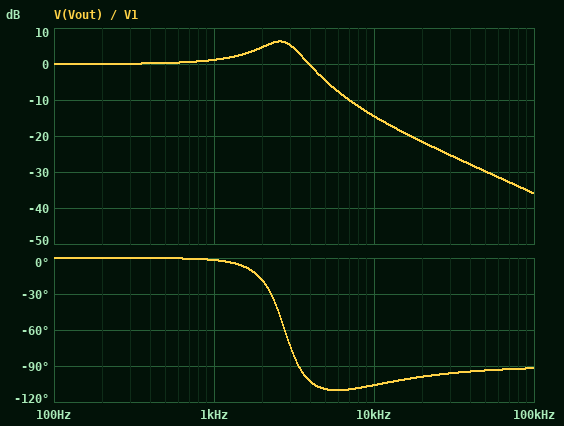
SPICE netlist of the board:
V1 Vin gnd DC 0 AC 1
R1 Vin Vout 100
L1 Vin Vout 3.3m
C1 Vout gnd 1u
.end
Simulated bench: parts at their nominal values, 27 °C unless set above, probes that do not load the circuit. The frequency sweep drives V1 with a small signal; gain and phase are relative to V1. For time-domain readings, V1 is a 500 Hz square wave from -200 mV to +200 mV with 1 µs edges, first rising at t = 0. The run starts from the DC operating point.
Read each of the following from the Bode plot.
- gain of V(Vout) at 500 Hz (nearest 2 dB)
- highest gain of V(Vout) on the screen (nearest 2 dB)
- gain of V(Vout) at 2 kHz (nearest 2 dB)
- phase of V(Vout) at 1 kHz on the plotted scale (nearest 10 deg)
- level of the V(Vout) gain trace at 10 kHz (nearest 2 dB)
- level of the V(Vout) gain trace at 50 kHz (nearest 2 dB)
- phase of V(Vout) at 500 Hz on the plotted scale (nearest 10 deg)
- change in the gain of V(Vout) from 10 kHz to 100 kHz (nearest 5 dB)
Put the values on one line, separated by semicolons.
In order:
0 dB; 6 dB; 4 dB; 0 deg; -14 dB; -30 dB; 0 deg; -20 dB
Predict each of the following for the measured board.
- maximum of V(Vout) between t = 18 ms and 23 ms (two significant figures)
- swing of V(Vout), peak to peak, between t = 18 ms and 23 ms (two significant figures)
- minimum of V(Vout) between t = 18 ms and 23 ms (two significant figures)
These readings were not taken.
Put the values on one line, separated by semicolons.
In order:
390 mV; 770 mV; -390 mV
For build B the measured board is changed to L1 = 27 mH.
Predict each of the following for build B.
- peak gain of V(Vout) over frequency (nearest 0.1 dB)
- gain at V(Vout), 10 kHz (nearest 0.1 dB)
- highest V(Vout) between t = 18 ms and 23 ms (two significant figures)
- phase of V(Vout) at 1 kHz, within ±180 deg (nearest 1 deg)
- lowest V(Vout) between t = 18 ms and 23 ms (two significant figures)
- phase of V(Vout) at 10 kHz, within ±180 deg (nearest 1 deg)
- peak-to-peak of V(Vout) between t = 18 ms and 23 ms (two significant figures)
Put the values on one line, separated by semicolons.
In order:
1.7 dB; -16.0 dB; 270 mV; -33 deg; -270 mV; -84 deg; 540 mV
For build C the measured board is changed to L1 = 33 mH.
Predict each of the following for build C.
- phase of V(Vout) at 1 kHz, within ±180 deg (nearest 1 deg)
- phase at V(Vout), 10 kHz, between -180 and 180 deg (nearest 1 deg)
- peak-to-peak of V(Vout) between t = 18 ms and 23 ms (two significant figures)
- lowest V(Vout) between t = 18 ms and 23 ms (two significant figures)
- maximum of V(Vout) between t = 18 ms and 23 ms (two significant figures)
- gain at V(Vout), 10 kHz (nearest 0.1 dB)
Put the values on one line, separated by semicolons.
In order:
-34 deg; -84 deg; 520 mV; -260 mV; 260 mV; -16.0 dB
